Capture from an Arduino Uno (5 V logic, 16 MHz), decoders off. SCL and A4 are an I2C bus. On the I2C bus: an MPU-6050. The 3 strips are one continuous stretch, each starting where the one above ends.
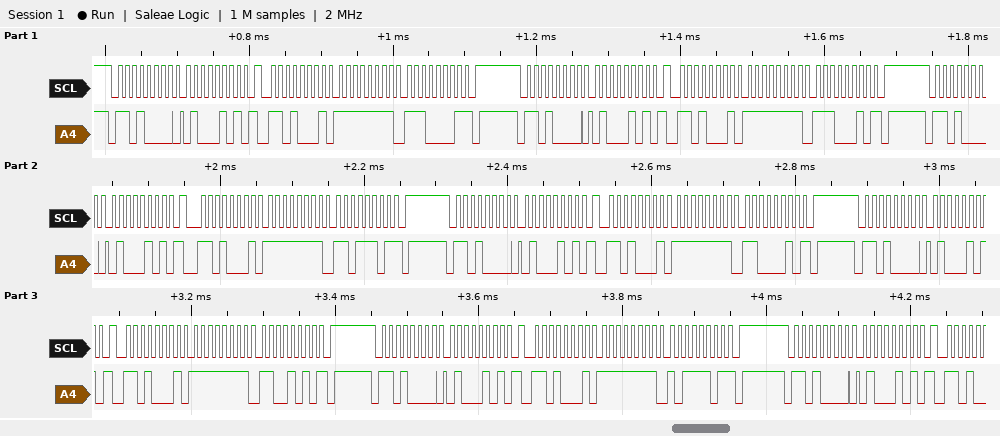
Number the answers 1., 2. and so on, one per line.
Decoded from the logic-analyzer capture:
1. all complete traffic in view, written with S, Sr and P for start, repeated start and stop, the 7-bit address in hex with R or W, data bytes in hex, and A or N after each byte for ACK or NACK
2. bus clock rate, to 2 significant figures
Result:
1. S 68W A 45 A Sr 68R A FF A E1 N P S 68W A 45 A Sr 68R A FF A E2 N P S 68W A 45 A Sr 68R A FF A DD N P S 68W A 45 A Sr 68R A FF A C2 N P S 68W A 45 A Sr 68R A FF A CA N P S 68W A 45 A Sr 68R A FF A BD N P S 68W A 45 A
2. 100 kHz
